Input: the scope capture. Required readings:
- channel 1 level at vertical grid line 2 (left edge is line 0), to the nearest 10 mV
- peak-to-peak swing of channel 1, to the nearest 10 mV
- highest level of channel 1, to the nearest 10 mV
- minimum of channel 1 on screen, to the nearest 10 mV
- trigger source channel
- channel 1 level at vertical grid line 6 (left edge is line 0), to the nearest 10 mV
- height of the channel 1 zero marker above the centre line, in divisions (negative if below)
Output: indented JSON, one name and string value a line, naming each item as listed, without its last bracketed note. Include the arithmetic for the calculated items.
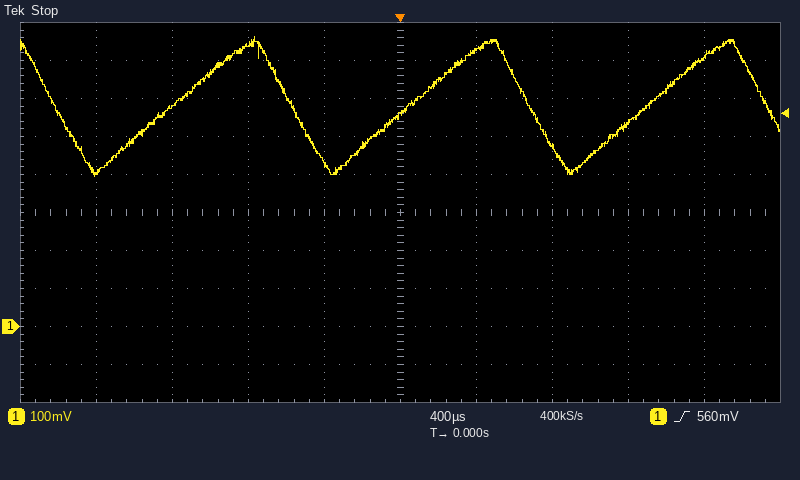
{
  "channel 1 level at vertical grid line 2 (left edge is line 0), to the nearest 10 mV": "580 mV",
  "peak-to-peak swing of channel 1, to the nearest 10 mV": "760 mV − (390 mV) = 370 mV",
  "highest level of channel 1, to the nearest 10 mV": "760 mV",
  "minimum of channel 1 on screen, to the nearest 10 mV": "390 mV",
  "trigger source channel": "channel 1",
  "channel 1 level at vertical grid line 6 (left edge is line 0), to the nearest 10 mV": "730 mV",
  "height of the channel 1 zero marker above the centre line, in divisions": "-3.0 div"
}
